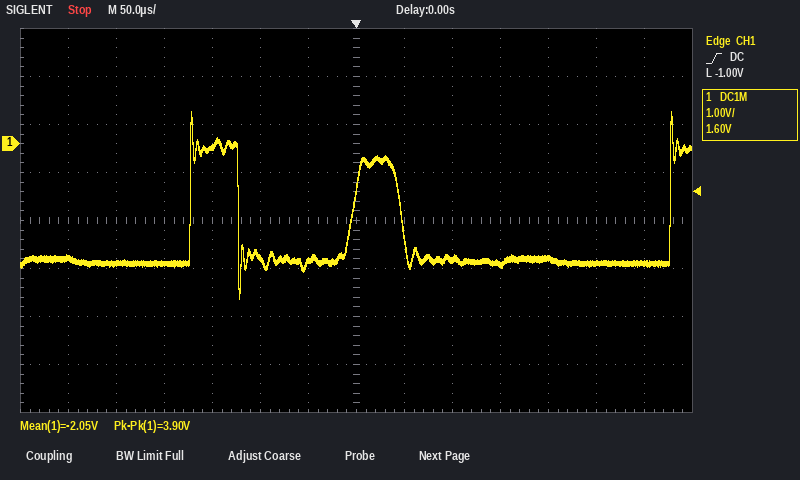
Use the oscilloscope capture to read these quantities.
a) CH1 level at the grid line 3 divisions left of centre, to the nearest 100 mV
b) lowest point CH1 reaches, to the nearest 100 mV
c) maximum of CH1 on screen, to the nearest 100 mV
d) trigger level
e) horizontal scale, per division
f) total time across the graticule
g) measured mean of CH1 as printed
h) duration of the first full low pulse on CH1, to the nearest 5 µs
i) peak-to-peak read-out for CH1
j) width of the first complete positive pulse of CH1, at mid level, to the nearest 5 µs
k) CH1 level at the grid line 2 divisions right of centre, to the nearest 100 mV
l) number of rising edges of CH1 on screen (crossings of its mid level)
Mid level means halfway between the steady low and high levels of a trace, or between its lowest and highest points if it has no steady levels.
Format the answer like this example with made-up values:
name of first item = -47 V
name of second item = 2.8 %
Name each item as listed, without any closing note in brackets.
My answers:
CH1 level at the grid line 3 divisions left of centre, to the nearest 100 mV = -100 mV
lowest point CH1 reaches, to the nearest 100 mV = -3.2 V
maximum of CH1 on screen, to the nearest 100 mV = 700 mV
trigger level = -1.00 V
horizontal scale, per division = 50 µs
total time across the graticule = 700 µs
measured mean of CH1 as printed = -2.05 V
duration of the first full low pulse on CH1, to the nearest 5 µs = 120 µs
peak-to-peak read-out for CH1 = 3.90 V
width of the first complete positive pulse of CH1, at mid level, to the nearest 5 µs = 50 µs
CH1 level at the grid line 2 divisions right of centre, to the nearest 100 mV = -2.4 V
number of rising edges of CH1 on screen = 3
